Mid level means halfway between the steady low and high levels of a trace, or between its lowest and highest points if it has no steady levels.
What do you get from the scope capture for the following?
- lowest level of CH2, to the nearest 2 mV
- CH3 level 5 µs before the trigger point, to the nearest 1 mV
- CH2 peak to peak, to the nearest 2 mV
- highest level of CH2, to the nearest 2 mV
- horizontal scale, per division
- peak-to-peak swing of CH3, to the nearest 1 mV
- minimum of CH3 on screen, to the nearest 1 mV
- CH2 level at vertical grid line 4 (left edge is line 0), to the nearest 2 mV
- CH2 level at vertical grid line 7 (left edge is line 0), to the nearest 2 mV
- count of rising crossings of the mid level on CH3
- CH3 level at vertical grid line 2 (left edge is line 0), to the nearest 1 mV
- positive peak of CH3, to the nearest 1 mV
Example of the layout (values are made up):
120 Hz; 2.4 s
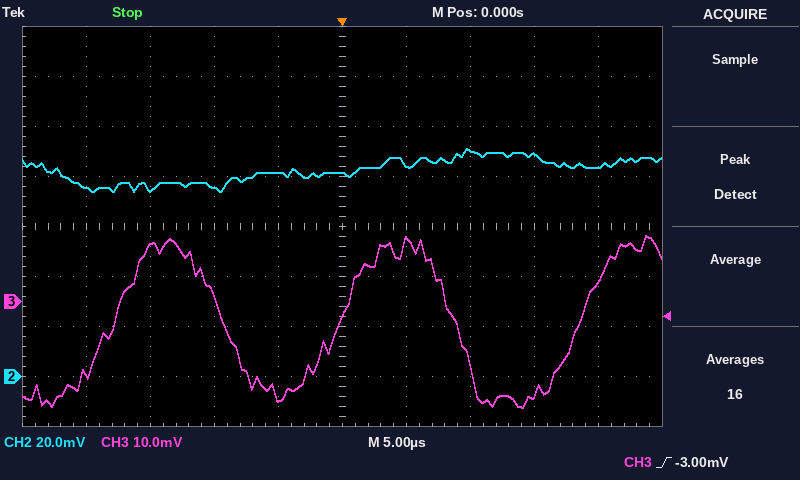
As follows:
74 mV; -19 mV; 18 mV; 92 mV; 5 µs; 34 mV; -21 mV; 82 mV; 90 mV; 3; 11 mV; 13 mV
